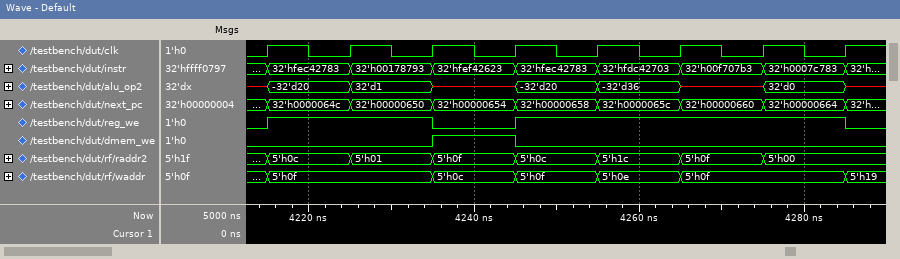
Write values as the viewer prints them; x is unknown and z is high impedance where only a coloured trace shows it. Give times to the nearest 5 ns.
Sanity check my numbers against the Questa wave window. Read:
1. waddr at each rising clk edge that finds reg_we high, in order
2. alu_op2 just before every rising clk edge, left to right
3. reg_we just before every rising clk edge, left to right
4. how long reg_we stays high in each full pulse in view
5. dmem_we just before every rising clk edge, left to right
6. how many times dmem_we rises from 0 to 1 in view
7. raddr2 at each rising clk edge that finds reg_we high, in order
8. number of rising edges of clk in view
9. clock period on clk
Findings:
5'h0f, 5'h0f, 5'h0f, 5'h0e, 5'h0f, 5'h0f
x, -32'd20, 32'd1, x, -32'd20, -32'd36, x, 32'd0
0 1 1 0 1 1 1 1
20 ns, 40 ns
0 0 0 1 0 0 0 0
1
5'h0c, 5'h01, 5'h0c, 5'h1c, 5'h0f, 5'h00
8
10 ns
